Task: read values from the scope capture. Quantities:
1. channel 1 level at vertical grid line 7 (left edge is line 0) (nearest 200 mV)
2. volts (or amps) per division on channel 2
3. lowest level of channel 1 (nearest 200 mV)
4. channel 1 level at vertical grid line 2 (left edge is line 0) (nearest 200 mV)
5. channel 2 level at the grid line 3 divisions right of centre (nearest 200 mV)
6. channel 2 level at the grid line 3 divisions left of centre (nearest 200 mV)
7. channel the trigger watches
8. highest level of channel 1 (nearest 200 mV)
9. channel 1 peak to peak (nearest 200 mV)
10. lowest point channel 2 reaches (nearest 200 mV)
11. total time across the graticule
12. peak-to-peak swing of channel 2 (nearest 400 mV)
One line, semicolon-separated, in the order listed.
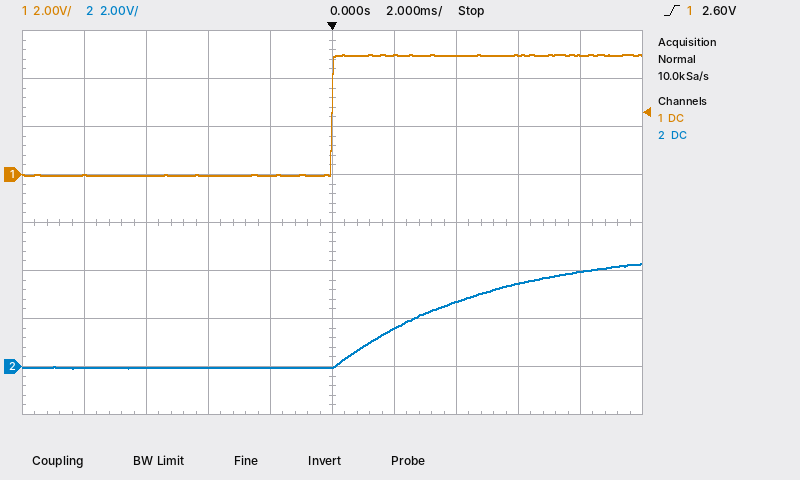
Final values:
5.0 V; 2 V; 0.0 V; 0.0 V; 3.4 V; 0.0 V; channel 1; 5.0 V; 5.0 V; 0.0 V; 20 ms; 4.4 V
